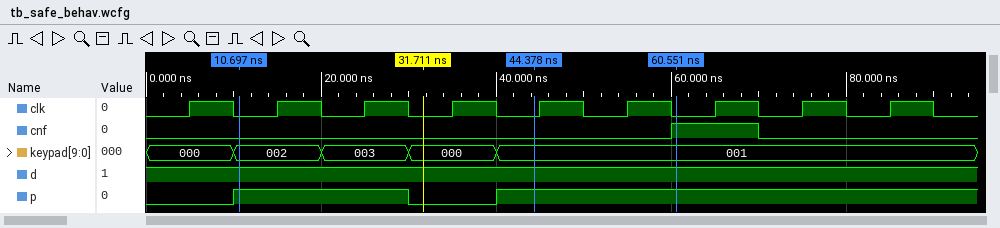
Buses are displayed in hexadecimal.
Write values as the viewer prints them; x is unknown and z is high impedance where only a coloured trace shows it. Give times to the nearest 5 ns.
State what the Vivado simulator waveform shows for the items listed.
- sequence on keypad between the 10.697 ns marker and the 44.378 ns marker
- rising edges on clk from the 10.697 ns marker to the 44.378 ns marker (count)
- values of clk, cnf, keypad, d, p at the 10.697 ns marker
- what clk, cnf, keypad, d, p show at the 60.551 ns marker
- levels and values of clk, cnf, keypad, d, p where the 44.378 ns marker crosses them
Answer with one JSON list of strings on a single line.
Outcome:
["002, 003, 000, 001", "3", "clk=0, cnf=0, keypad=002, d=1, p=1", "clk=0, cnf=1, keypad=001, d=1, p=1", "clk=0, cnf=0, keypad=001, d=1, p=1"]
